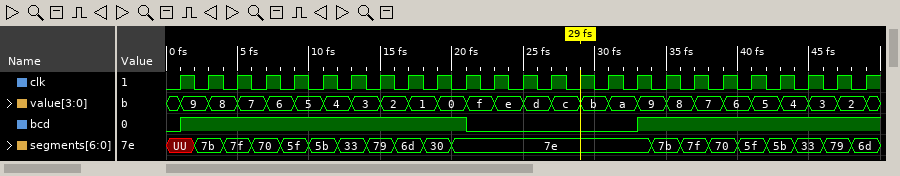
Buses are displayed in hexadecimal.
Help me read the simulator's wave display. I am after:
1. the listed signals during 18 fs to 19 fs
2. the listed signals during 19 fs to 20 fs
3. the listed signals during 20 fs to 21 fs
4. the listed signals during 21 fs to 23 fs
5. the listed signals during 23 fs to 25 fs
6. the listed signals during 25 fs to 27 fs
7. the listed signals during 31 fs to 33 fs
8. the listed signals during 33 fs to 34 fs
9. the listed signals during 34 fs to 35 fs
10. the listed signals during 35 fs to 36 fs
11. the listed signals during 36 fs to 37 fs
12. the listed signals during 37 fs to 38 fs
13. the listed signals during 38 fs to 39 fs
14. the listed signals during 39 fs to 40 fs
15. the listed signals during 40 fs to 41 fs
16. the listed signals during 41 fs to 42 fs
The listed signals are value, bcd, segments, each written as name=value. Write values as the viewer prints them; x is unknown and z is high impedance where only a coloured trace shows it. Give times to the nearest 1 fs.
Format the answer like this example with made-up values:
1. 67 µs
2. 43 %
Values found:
1. value=1, bcd=1, segments=30
2. value=0, bcd=1, segments=30
3. value=0, bcd=1, segments=7e
4. value=f, bcd=0, segments=7e
5. value=e, bcd=0, segments=7e
6. value=d, bcd=0, segments=7e
7. value=a, bcd=0, segments=7e
8. value=9, bcd=1, segments=7e
9. value=9, bcd=1, segments=7b
10. value=8, bcd=1, segments=7b
11. value=8, bcd=1, segments=7f
12. value=7, bcd=1, segments=7f
13. value=7, bcd=1, segments=70
14. value=6, bcd=1, segments=70
15. value=6, bcd=1, segments=5f
16. value=5, bcd=1, segments=5f
